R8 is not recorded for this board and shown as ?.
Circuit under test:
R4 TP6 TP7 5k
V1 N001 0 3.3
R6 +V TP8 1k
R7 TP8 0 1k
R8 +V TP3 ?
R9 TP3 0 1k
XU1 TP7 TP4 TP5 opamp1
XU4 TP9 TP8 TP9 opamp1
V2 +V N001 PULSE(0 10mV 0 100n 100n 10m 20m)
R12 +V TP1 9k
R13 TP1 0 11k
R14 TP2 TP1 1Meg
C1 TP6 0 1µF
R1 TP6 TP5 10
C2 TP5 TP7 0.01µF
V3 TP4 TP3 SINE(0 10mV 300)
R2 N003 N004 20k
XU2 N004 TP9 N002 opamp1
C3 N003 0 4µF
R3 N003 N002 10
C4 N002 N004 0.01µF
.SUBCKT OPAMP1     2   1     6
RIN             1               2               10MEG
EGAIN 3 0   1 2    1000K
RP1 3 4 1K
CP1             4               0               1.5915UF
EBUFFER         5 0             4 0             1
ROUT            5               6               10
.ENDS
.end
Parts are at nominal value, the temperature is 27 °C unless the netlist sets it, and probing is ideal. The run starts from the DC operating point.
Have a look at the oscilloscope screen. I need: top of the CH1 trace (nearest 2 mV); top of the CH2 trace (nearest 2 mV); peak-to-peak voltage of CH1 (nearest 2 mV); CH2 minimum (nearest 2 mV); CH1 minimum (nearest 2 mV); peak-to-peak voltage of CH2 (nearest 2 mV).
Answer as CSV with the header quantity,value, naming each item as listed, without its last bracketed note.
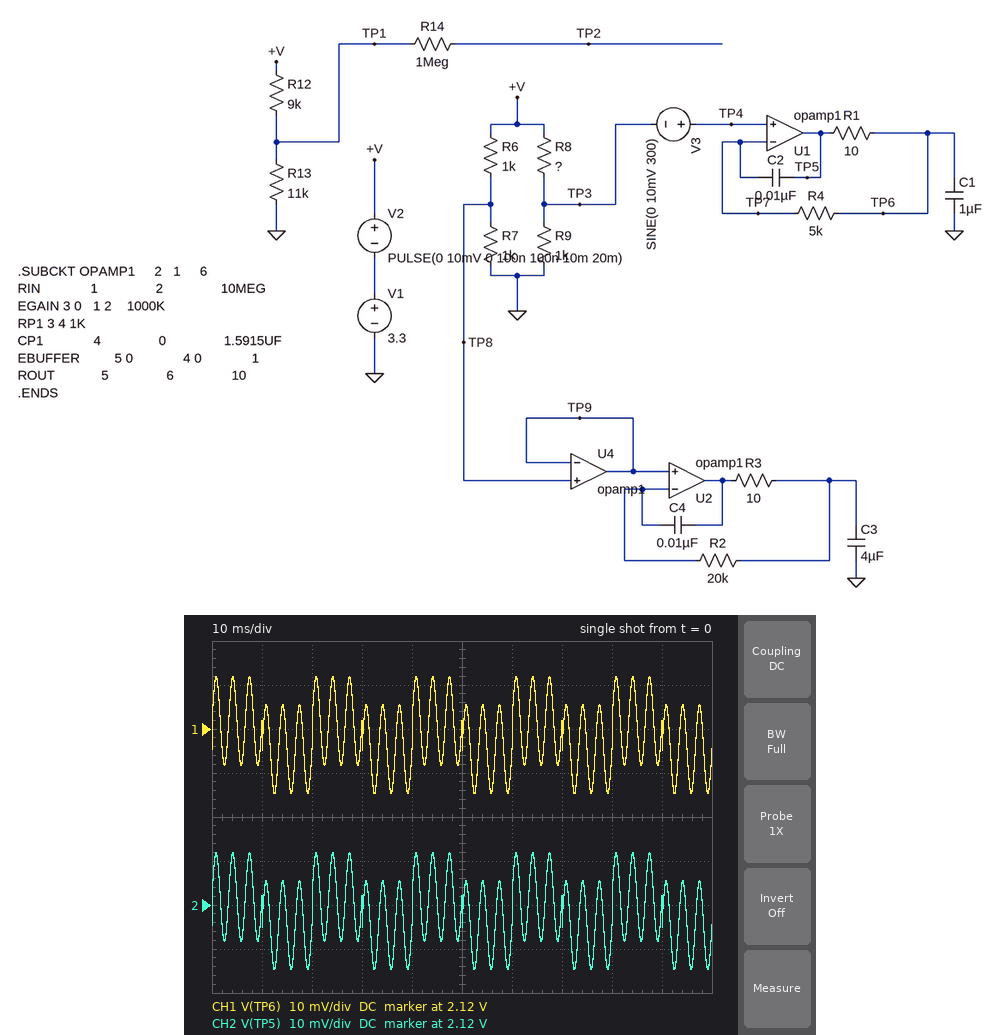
quantity,value
top of the CH1 trace,2.132 V
top of the CH2 trace,2.132 V
peak-to-peak voltage of CH1,26 mV
CH2 minimum,2.106 V
CH1 minimum,2.106 V
peak-to-peak voltage of CH2,26 mV
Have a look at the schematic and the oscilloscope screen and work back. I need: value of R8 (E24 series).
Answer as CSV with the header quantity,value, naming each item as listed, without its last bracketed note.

quantity,value
value of R8,560 Ω
